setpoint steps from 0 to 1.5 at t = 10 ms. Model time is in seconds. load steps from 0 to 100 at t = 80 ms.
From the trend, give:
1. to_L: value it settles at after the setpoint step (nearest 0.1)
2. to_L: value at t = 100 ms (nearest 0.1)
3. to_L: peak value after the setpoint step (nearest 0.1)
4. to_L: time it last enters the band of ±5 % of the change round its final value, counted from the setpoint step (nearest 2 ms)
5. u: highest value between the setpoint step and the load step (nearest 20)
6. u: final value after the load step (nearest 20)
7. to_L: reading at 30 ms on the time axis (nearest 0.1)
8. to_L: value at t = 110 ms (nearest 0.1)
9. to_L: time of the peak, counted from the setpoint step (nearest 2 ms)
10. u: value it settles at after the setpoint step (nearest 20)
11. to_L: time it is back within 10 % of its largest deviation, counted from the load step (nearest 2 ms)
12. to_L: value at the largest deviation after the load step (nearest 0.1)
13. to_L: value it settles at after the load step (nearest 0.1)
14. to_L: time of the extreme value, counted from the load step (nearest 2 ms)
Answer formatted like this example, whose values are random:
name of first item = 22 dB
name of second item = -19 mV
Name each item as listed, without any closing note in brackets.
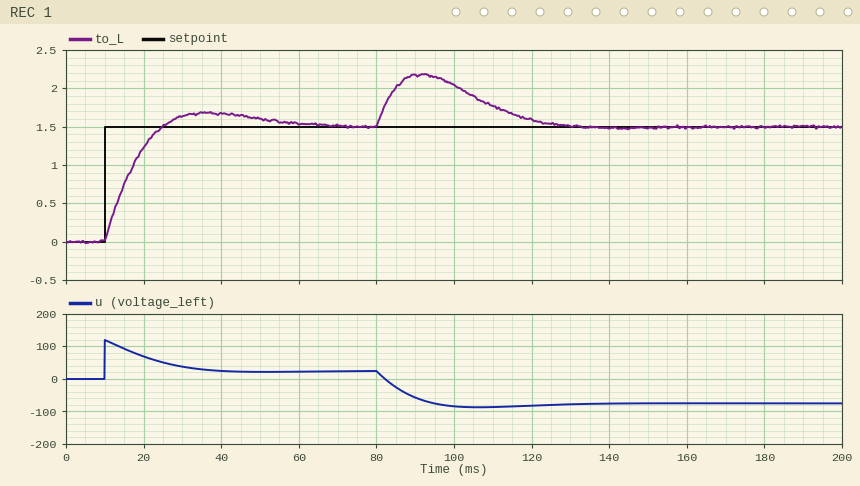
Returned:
to_L: value it settles at after the setpoint step = 1.5
to_L: value at t = 100 ms = 2.0
to_L: peak value after the setpoint step = 1.7
to_L: time it last enters the band of ±5 % of the change round its final value, counted from the setpoint step = 44 ms
u: highest value between the setpoint step and the load step = 120
u: final value after the load step = -80
to_L: reading at 30 ms on the time axis = 1.6
to_L: value at t = 110 ms = 1.8
to_L: time of the peak, counted from the setpoint step = 26 ms
u: value it settles at after the setpoint step = 20
to_L: time it is back within 10 % of its largest deviation, counted from the load step = 42 ms
to_L: value at the largest deviation after the load step = 2.2
to_L: value it settles at after the load step = 1.5
to_L: time of the extreme value, counted from the load step = 12 ms
